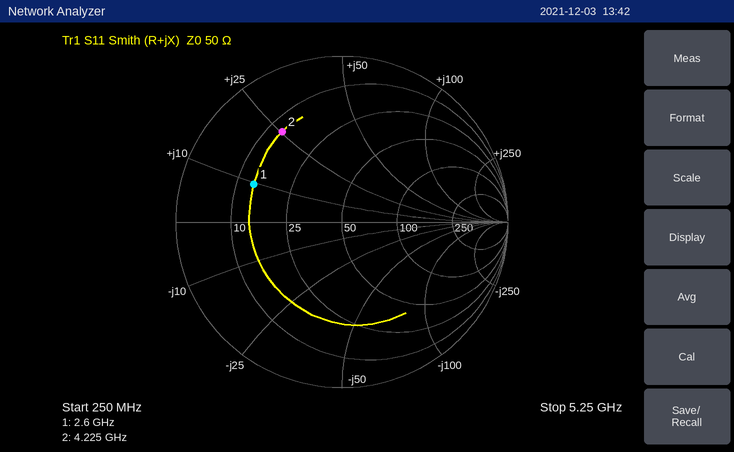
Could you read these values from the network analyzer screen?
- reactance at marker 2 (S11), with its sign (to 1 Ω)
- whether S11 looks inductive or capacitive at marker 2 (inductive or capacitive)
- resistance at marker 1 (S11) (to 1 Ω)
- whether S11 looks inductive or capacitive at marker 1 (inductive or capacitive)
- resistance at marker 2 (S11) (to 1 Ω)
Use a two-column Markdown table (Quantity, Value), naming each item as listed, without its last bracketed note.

| Quantity | Value |
|---|---|
| reactance at marker 2 (S11), with its sign | +25 Ω |
| whether S11 looks inductive or capacitive at marker 2 | inductive |
| resistance at marker 1 (S11) | 14 Ω |
| whether S11 looks inductive or capacitive at marker 1 | inductive |
| resistance at marker 2 (S11) | 13 Ω |
